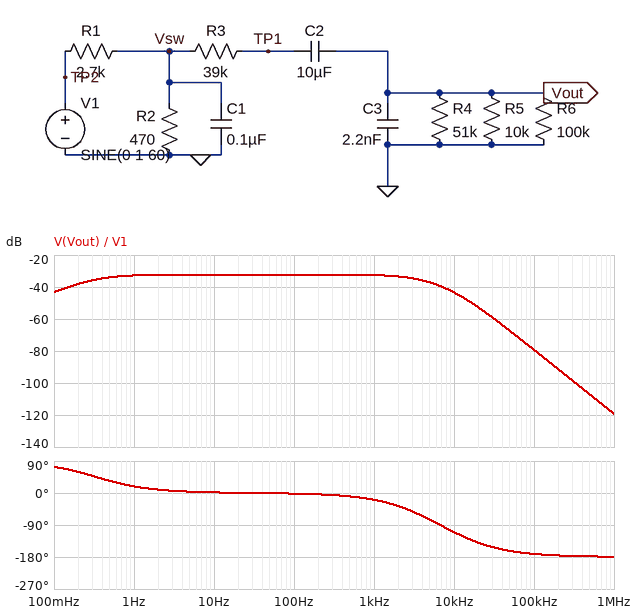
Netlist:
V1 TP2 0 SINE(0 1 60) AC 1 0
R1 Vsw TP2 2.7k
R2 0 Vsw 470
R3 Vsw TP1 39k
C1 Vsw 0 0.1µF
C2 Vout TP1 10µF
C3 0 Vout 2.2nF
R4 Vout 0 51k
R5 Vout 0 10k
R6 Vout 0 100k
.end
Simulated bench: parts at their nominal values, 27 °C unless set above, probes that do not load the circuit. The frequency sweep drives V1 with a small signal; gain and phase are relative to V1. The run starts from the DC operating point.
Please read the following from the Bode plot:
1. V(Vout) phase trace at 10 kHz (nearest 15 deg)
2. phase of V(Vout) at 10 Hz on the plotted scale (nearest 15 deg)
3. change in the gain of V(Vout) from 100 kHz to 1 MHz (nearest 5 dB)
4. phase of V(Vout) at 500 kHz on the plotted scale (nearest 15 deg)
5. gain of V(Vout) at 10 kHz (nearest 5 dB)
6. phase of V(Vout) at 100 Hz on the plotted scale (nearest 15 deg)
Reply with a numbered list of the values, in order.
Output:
1. -105 deg
2. 0 deg
3. -40 dB
4. -180 deg
5. -45 dB
6. 0 deg
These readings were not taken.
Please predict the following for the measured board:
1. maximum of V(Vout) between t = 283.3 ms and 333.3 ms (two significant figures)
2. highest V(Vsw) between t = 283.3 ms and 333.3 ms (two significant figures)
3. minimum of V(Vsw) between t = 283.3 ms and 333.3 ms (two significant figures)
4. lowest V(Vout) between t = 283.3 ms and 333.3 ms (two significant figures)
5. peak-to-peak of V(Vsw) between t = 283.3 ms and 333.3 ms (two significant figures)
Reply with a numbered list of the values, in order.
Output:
1. 24 mV
2. 150 mV
3. -150 mV
4. -24 mV
5. 290 mV
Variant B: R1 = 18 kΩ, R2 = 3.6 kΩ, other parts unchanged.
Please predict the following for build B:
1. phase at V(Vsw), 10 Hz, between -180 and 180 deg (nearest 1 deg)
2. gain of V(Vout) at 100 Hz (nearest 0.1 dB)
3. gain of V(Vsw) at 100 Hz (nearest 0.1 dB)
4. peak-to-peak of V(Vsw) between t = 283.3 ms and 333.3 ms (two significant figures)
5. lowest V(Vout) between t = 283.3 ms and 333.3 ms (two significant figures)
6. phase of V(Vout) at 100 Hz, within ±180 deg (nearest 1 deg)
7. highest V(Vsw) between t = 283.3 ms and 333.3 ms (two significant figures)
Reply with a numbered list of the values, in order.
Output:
1. -1 deg
2. -31.9 dB
3. -16.2 dB
4. 310 mV
5. -26 mV
6. -10 deg
7. 160 mV
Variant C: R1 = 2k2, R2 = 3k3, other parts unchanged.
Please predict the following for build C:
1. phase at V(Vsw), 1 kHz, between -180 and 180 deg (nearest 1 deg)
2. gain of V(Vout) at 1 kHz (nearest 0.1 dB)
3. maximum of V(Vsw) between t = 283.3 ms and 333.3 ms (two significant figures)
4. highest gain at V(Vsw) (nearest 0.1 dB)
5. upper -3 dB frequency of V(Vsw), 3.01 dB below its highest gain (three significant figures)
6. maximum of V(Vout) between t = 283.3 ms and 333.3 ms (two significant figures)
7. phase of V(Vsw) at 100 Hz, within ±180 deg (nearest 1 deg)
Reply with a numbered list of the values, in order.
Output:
1. -39 deg
2. -22.5 dB
3. 580 mV
4. -4.4 dB
5. 1.17 kHz
6. 96 mV
7. -5 deg
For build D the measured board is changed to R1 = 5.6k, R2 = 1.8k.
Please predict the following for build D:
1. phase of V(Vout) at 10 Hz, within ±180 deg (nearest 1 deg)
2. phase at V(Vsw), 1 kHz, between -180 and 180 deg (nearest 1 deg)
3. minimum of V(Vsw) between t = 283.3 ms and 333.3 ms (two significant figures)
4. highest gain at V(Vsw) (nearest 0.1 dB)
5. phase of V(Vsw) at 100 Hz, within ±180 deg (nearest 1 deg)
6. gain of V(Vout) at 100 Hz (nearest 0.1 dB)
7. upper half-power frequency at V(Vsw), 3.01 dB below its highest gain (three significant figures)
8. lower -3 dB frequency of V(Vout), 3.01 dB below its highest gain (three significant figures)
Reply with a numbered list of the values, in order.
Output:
1. 1 deg
2. -40 deg
3. -240 mV
4. -12.3 dB
5. -5 deg
6. -28.2 dB
7. 1.13 kHz
8. 331 mHz
